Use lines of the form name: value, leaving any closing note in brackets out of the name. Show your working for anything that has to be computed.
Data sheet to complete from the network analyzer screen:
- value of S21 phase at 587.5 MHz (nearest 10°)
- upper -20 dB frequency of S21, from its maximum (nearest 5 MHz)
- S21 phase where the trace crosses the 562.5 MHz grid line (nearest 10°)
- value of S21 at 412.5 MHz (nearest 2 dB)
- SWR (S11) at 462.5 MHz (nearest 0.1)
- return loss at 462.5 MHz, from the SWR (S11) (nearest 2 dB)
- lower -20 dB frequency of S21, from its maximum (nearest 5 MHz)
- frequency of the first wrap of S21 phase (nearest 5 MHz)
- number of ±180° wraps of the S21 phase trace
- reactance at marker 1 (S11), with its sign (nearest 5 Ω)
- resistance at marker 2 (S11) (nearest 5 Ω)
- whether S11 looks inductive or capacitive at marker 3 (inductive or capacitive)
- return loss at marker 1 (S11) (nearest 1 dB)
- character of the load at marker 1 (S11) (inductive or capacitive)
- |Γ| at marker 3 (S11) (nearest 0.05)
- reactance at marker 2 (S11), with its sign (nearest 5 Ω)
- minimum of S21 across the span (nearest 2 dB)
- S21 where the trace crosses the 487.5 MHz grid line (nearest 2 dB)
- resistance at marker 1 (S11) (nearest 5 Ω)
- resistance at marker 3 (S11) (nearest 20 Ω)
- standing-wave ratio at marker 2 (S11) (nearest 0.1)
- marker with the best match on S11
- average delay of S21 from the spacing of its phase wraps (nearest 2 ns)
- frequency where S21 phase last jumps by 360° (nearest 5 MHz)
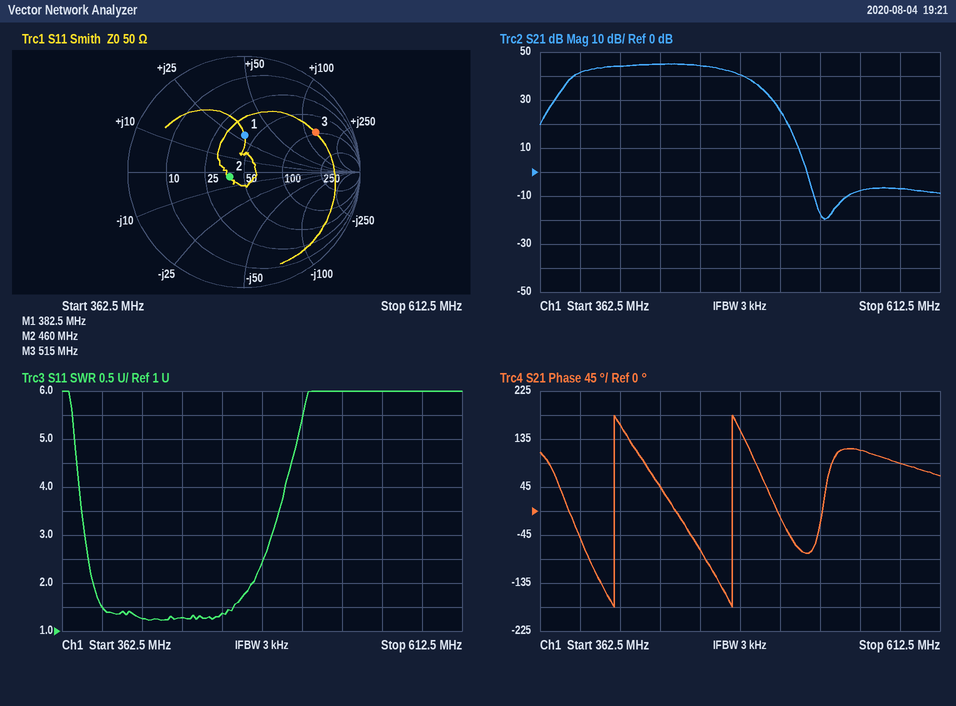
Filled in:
value of S21 phase at 587.5 MHz: 90°
upper -20 dB frequency of S21, from its maximum: 515 MHz
S21 phase where the trace crosses the 562.5 MHz grid line: 110°
value of S21 at 412.5 MHz: 44 dB
SWR (S11) at 462.5 MHz: 1.4
return loss at 462.5 MHz, from the SWR (S11): −20 log10((1.4 − 1)/(1.4 + 1)) ≈ 16 dB
lower -20 dB frequency of S21, from its maximum: 365 MHz
frequency of the first wrap of S21 phase: 410 MHz
number of ±180° wraps of the S21 phase trace: 2
reactance at marker 1 (S11), with its sign: +30 Ω
resistance at marker 2 (S11): 40 Ω
whether S11 looks inductive or capacitive at marker 3: inductive
return loss at marker 1 (S11): 10 dB
character of the load at marker 1 (S11): inductive
|Γ| at marker 3 (S11): 0.70
reactance at marker 2 (S11), with its sign: -5 Ω
minimum of S21 across the span: -20 dB
S21 where the trace crosses the 487.5 MHz grid line: 40 dB
resistance at marker 1 (S11): 40 Ω
resistance at marker 3 (S11): 100 Ω
standing-wave ratio at marker 2 (S11): 1.3
marker with the best match on S11: marker 2
average delay of S21 from the spacing of its phase wraps: 1 cycle / (485 MHz − 410 MHz) ≈ 13.3 ns, so 14 ns to the nearest 2 ns
frequency where S21 phase last jumps by 360°: 485 MHz
